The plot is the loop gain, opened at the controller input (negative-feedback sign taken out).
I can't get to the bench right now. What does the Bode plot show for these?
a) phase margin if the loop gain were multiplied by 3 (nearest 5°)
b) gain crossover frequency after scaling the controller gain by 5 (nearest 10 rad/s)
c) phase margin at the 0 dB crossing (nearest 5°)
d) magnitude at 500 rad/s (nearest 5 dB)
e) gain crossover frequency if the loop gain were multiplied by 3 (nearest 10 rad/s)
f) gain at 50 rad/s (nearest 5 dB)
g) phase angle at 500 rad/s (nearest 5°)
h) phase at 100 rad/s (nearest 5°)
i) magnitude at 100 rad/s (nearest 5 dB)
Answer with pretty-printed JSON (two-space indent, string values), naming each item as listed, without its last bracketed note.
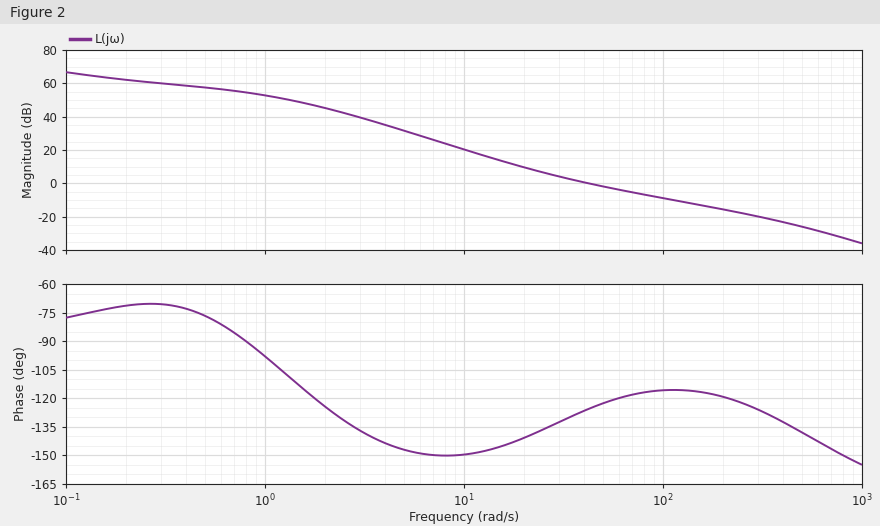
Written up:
{
  "phase margin if the loop gain were multiplied by 3": "65°",
  "gain crossover frequency after scaling the controller gain by 5": "170 rad/s",
  "phase margin at the 0 dB crossing": "55°",
  "magnitude at 500 rad/s": "-25 dB",
  "gain crossover frequency if the loop gain were multiplied by 3": "110 rad/s",
  "gain at 50 rad/s": "0 dB",
  "phase angle at 500 rad/s": "-140°",
  "phase at 100 rad/s": "-115°",
  "magnitude at 100 rad/s": "-10 dB"
}
